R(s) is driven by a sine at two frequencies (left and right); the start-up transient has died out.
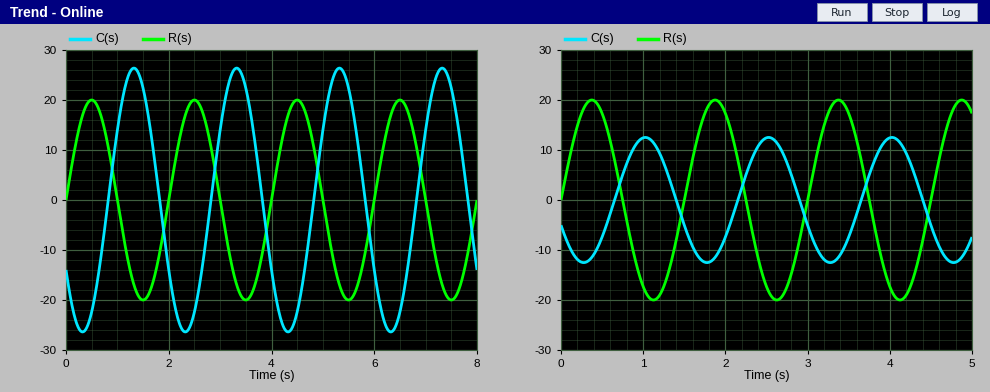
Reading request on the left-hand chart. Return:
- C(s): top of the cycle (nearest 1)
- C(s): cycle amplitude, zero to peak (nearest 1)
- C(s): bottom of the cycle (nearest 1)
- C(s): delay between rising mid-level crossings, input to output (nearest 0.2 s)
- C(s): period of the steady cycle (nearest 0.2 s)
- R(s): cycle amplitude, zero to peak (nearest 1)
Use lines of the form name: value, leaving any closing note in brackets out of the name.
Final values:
C(s): top of the cycle: 26
C(s): cycle amplitude, zero to peak: 26
C(s): bottom of the cycle: -26
C(s): delay between rising mid-level crossings, input to output: 0.8 s
C(s): period of the steady cycle: 2.0 s
R(s): cycle amplitude, zero to peak: 20
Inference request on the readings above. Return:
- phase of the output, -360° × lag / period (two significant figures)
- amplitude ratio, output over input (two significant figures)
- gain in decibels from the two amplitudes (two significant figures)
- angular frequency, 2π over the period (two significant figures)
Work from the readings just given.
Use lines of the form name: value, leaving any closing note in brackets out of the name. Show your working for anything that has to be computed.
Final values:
phase of the output, -360° × lag / period: -360 × 0.8 / 2 = -140°
amplitude ratio, output over input: 26 / 20 = 1.3
gain in decibels from the two amplitudes: 20 log10(26 / 20) = 2.3 dB
angular frequency, 2π over the period: 2π / 2 = 3.1 rad/s
